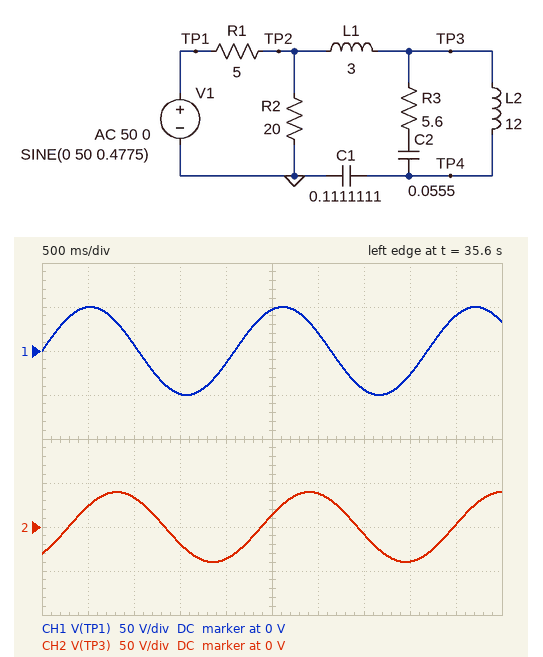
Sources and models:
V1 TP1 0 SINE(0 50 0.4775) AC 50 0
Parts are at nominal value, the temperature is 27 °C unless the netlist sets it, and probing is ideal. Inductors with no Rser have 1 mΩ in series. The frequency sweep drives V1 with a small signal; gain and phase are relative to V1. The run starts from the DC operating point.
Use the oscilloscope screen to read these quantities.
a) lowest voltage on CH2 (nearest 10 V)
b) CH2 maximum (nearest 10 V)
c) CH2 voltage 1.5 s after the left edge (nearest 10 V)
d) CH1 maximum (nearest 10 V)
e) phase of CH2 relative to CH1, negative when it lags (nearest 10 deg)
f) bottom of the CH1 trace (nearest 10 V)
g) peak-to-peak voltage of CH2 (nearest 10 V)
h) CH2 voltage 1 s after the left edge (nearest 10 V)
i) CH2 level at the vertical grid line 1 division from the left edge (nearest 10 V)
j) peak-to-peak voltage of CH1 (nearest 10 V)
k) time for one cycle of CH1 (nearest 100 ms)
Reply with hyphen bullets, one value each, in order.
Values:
- -40 V
- 40 V
- -20 V
- 50 V
- -50 deg
- -50 V
- 80 V
- 30 V
- 20 V
- 100 V
- 2.1 s
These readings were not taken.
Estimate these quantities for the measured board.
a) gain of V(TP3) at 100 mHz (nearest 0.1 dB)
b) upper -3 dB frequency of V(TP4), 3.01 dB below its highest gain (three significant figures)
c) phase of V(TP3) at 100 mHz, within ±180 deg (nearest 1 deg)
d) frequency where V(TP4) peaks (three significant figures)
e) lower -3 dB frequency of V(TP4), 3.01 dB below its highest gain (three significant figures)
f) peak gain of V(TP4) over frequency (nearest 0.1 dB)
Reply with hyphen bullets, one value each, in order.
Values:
- -3.6 dB
- 116 mHz
- -54 deg
- 103 mHz
- 85.1 mHz
- 7.0 dB
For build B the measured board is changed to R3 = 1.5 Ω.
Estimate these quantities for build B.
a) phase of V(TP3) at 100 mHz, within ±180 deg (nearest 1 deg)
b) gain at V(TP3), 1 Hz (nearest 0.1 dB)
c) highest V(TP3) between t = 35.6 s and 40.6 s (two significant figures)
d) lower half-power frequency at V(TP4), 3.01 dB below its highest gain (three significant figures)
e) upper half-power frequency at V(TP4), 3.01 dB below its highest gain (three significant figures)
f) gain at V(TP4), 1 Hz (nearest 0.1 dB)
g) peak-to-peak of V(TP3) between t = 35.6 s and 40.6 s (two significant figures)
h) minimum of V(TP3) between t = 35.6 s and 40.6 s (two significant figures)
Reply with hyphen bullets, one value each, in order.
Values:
- -59 deg
- -12.4 dB
- 66 V
- 89.4 mHz
- 116 mHz
- -22.6 dB
- 130 V
- -66 V
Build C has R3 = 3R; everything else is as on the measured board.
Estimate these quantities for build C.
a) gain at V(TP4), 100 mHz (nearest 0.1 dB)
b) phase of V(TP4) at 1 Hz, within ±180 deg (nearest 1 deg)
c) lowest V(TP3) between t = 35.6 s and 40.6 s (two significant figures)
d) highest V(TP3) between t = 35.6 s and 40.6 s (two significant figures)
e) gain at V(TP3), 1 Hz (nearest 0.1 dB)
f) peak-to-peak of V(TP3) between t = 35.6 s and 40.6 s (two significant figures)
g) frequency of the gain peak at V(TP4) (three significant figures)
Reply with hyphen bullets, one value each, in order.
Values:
- 7.3 dB
- -154 deg
- -51 V
- 51 V
- -11.6 dB
- 100 V
- 104 mHz
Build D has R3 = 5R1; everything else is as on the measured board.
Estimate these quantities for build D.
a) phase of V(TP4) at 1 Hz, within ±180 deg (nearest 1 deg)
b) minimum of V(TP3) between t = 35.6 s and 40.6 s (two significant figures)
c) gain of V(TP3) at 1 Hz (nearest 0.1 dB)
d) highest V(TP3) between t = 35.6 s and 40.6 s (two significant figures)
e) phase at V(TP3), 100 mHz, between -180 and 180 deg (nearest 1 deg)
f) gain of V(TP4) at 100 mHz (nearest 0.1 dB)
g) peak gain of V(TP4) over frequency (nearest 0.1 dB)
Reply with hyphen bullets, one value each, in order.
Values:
- -147 deg
- -41 V
- -10.2 dB
- 41 V
- -55 deg
- 6.9 dB
- 7.1 dB
